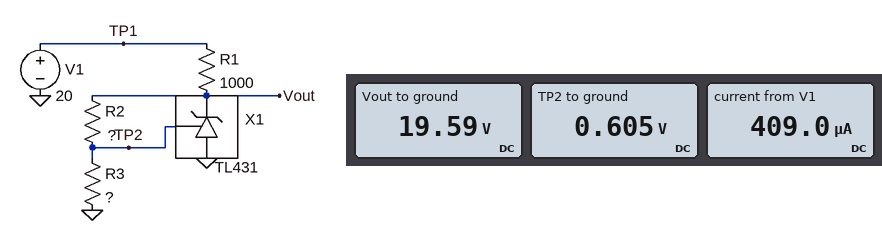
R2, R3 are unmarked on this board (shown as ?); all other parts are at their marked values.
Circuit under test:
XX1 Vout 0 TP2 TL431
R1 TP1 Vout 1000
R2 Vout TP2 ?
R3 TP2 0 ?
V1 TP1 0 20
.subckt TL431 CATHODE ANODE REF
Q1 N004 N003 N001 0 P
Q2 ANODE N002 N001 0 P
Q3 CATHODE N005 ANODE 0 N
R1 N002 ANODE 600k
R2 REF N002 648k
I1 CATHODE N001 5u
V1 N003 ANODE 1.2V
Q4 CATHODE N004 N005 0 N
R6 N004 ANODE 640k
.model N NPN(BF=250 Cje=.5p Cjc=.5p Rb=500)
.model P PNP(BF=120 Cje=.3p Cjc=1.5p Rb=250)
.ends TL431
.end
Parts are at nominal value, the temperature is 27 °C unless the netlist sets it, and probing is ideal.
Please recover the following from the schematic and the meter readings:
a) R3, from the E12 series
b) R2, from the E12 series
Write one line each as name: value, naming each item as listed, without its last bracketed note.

R3, from the E12 series: 1.5 kΩ
R2, from the E12 series: 47 kΩ
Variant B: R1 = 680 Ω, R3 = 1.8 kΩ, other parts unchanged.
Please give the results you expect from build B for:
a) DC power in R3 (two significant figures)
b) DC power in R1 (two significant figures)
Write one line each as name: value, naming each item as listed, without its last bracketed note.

DC power in R3: 290 µW
DC power in R1: 110 µW
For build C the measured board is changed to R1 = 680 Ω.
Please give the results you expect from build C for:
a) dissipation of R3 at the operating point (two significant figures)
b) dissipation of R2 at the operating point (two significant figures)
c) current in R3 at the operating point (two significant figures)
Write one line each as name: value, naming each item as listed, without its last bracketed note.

dissipation of R3 at the operating point: 250 µW
dissipation of R2 at the operating point: 7.8 mW
current in R3 at the operating point: 410 µA
